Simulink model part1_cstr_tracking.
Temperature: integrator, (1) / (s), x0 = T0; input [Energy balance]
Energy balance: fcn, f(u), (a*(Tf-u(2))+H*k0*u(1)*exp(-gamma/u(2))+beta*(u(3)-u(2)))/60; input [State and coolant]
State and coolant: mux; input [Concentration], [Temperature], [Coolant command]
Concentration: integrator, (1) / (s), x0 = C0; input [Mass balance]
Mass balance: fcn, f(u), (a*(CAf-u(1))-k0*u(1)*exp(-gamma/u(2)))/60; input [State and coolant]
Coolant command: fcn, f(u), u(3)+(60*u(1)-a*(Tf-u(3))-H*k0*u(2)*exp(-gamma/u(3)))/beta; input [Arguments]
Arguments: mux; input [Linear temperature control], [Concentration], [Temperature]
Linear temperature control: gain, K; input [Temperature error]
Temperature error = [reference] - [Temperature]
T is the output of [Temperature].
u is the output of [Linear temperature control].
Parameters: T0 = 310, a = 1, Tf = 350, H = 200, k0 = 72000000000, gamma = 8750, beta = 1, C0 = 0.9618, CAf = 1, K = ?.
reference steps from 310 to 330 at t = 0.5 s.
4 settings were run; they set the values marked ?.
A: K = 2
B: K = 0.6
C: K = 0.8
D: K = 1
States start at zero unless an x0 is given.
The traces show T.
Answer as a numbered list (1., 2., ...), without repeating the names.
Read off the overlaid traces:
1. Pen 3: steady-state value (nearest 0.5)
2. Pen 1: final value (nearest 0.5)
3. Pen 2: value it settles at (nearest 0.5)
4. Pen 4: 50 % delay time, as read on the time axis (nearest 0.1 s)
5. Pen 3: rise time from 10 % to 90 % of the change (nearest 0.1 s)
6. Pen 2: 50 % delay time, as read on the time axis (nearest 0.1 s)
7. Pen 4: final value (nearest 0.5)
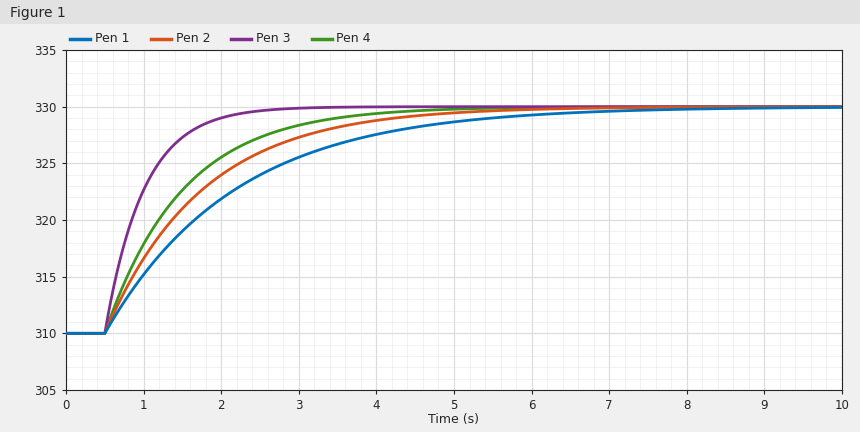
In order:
1. 330.0
2. 330.0
3. 330.0
4. 1.2 s
5. 1.1 s
6. 1.4 s
7. 330.0
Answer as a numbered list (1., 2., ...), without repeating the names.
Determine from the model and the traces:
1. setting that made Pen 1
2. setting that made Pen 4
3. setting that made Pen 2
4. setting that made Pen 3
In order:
1. B
2. D
3. C
4. A
